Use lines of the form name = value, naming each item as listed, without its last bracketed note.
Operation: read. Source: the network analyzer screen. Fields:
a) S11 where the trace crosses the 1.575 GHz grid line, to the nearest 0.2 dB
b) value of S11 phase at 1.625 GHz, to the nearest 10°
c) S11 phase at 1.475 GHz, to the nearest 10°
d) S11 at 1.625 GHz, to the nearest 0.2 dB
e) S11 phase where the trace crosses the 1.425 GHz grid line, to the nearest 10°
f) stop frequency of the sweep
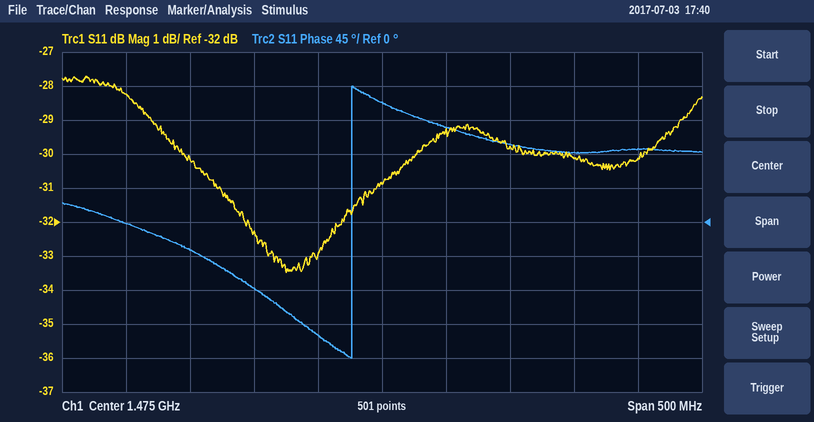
S11 where the trace crosses the 1.575 GHz grid line, to the nearest 0.2 dB = -29.8 dB
value of S11 phase at 1.625 GHz, to the nearest 10° = 90°
S11 phase at 1.475 GHz, to the nearest 10° = 160°
S11 at 1.625 GHz, to the nearest 0.2 dB = -30.2 dB
S11 phase where the trace crosses the 1.425 GHz grid line, to the nearest 10° = -150°
stop frequency of the sweep = 1.725 GHz
